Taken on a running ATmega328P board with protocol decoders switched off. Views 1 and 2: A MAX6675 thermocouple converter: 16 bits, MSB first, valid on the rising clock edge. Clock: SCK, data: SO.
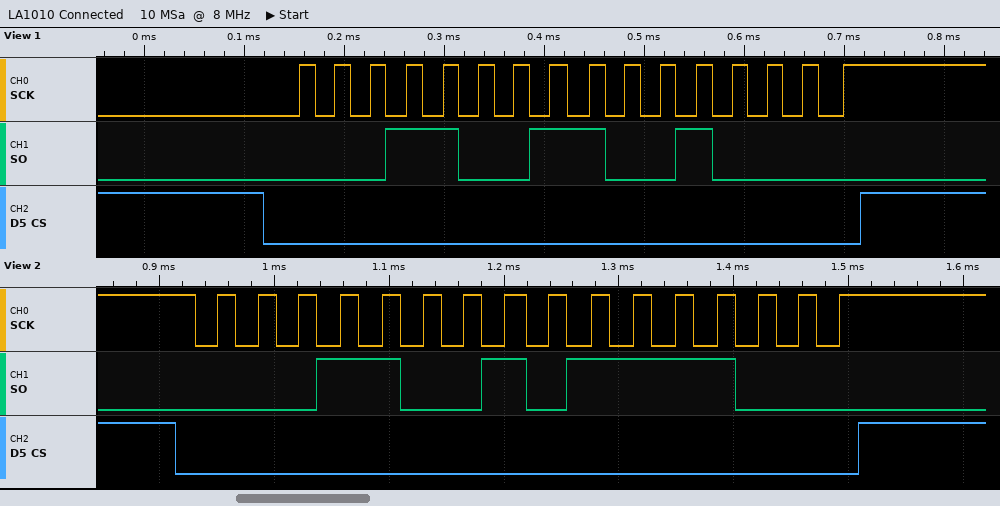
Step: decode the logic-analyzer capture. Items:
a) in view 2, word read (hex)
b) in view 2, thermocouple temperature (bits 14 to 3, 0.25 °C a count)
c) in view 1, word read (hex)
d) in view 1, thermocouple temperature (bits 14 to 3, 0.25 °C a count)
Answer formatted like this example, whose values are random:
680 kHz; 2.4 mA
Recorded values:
0x1978; 203.75 °C; 0x1990; 204.50 °C
